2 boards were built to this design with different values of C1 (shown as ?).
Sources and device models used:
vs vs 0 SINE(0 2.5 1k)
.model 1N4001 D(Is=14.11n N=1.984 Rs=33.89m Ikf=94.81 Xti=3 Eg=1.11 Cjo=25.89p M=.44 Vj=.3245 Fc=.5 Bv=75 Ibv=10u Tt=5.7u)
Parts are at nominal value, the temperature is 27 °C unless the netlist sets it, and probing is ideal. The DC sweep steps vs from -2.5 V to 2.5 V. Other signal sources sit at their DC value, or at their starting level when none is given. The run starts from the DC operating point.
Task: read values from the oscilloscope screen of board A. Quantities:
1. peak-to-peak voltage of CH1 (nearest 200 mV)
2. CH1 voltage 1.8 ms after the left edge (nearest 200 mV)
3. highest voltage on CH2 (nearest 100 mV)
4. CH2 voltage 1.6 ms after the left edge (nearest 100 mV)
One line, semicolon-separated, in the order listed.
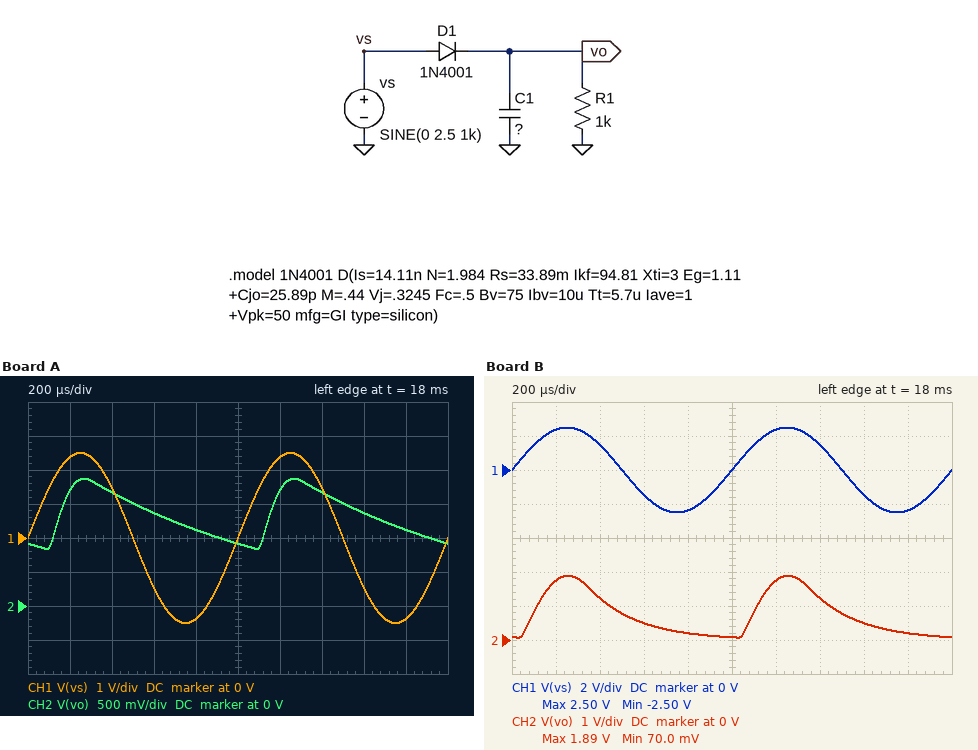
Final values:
5.0 V; -2.4 V; 1.9 V; 1.4 V
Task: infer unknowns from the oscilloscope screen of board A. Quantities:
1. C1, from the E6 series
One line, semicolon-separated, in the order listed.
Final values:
1 µF
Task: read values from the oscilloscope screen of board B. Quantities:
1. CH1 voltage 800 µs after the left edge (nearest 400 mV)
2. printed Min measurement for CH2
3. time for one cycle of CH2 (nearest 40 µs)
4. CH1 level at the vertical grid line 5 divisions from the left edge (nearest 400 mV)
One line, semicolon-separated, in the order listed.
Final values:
-2.4 V; 70.0 mV; 1.00 ms; 0 V
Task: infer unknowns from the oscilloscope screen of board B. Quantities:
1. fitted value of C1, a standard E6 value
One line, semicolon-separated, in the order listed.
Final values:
220 nF
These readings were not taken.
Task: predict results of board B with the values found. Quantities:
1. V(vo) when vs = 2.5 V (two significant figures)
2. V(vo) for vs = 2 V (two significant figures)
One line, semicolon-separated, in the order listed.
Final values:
1.9 V; 1.4 V
